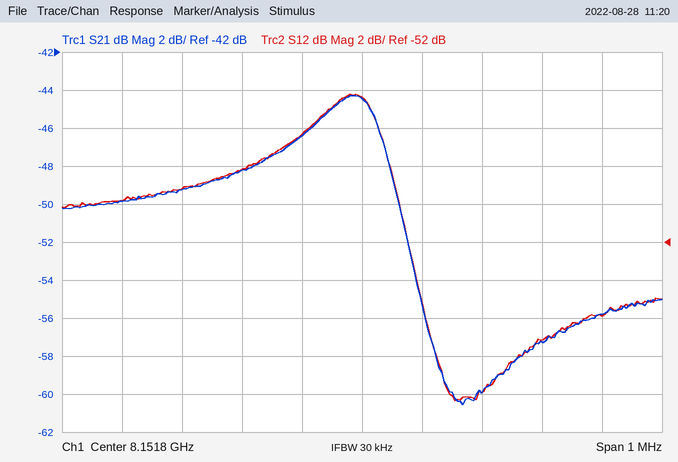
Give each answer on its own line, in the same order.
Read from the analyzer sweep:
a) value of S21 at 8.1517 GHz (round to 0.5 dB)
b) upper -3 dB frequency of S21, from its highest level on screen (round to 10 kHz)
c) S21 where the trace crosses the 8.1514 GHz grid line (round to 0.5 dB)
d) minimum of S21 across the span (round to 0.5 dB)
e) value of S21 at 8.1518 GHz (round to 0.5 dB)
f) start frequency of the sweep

-46.5 dB
8.15184 GHz
-50.0 dB
-60.5 dB
-44.5 dB
8.1513 GHz
